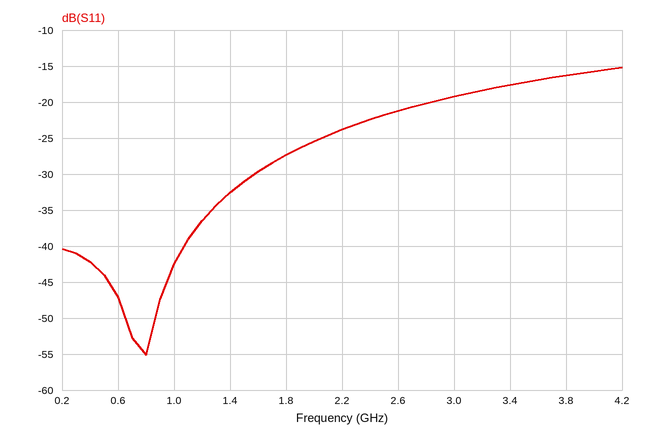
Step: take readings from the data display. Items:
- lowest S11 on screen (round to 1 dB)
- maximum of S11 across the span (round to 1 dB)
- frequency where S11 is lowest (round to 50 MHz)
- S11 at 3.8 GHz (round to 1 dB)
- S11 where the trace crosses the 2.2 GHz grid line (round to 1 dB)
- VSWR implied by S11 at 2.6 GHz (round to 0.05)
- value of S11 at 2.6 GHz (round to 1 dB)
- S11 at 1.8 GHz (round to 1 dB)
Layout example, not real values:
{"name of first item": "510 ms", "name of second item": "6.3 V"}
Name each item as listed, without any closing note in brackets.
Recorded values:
{"lowest S11 on screen": "-55 dB", "maximum of S11 across the span": "-15 dB", "frequency where S11 is lowest": "800 MHz", "S11 at 3.8 GHz": "-16 dB", "S11 where the trace crosses the 2.2 GHz grid line": "-24 dB", "VSWR implied by S11 at 2.6 GHz": "1.20", "value of S11 at 2.6 GHz": "-21 dB", "S11 at 1.8 GHz": "-27 dB"}
